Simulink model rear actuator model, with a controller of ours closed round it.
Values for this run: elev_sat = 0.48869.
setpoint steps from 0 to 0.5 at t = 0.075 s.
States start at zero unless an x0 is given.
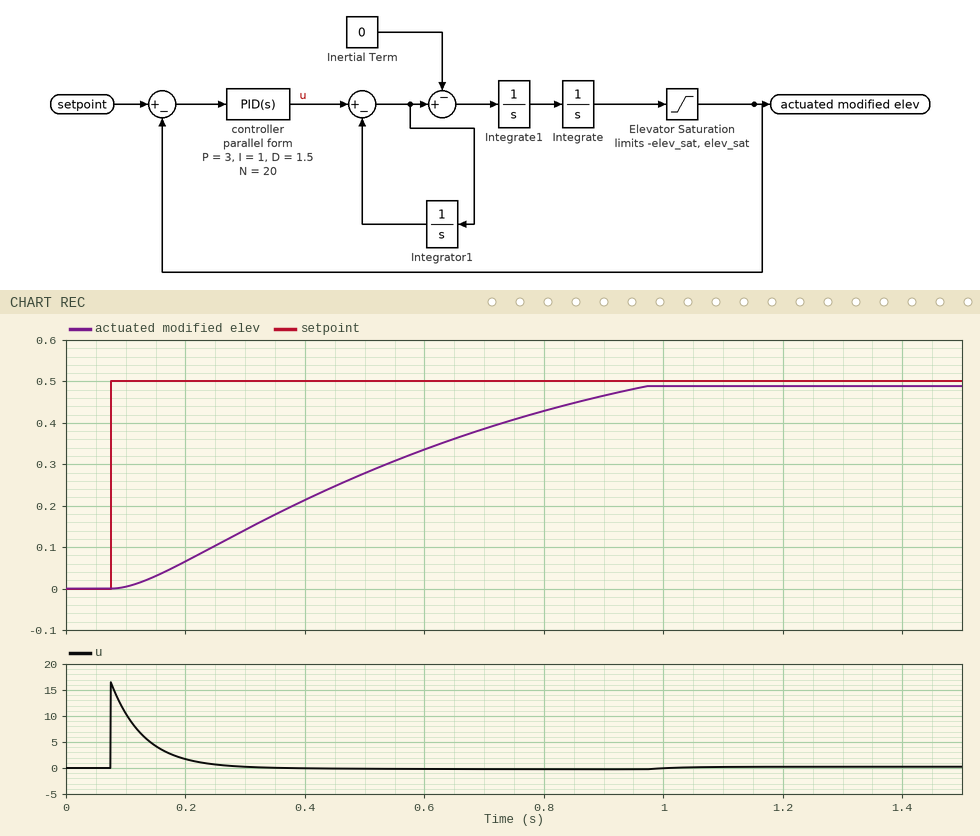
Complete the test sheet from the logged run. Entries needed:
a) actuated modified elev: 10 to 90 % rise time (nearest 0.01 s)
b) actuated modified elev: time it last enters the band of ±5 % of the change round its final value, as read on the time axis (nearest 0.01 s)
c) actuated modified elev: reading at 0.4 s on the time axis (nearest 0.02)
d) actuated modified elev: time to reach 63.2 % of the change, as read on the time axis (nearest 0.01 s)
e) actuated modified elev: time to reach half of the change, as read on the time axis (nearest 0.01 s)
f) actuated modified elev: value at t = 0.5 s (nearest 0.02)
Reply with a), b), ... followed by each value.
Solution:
a) 0.65 s
b) 0.90 s
c) 0.22
d) 0.55 s
e) 0.45 s
f) 0.28
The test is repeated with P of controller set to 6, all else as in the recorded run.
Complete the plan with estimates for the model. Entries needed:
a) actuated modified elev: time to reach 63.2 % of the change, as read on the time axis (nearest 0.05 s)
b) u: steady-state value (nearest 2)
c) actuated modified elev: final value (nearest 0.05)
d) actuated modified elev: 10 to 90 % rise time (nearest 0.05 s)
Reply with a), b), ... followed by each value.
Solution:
a) 0.45 s
b) 0
c) 0.50
d) 0.45 s
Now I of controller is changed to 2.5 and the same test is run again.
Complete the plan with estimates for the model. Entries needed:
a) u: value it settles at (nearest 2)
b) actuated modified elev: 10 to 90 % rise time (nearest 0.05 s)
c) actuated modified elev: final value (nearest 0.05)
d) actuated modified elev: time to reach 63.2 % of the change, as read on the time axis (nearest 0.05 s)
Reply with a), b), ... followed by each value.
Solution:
a) 0
b) 0.60 s
c) 0.50
d) 0.55 s
